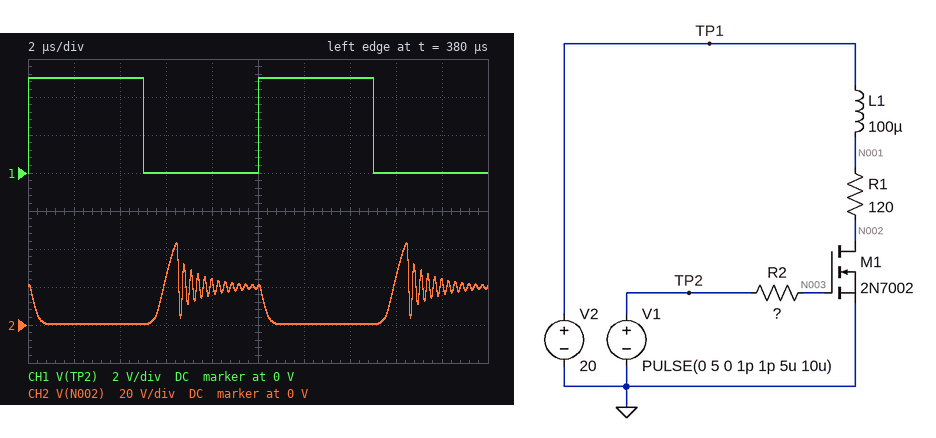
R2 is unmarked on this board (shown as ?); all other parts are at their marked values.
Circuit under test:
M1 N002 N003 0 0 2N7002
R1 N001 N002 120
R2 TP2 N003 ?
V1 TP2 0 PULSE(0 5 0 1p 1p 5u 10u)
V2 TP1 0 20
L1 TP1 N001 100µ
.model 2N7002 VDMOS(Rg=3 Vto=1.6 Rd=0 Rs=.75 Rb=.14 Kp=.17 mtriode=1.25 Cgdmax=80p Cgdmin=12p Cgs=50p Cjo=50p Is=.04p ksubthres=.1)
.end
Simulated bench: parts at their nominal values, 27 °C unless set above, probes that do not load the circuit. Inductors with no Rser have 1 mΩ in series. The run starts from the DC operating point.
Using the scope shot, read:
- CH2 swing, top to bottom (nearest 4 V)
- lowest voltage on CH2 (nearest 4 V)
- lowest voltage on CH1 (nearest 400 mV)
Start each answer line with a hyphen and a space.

- 44 V
- 0 V
- 0 V
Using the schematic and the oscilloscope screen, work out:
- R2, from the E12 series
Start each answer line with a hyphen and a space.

- 3.9 kΩ
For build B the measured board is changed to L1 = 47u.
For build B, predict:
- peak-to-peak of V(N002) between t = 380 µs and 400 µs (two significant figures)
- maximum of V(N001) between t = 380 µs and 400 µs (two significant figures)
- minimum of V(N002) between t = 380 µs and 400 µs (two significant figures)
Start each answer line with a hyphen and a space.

- 31 V
- 33 V
- 370 mV
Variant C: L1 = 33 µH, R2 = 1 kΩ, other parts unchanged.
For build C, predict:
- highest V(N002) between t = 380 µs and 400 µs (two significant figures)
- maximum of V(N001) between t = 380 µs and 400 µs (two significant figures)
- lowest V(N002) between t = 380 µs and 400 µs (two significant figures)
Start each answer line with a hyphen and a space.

- 48 V
- 49 V
- 280 mV
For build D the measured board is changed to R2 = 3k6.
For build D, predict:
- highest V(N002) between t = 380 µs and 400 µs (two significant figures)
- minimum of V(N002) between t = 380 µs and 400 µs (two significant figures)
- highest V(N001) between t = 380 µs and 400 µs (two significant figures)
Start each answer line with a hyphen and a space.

- 45 V
- 310 mV
- 46 V
